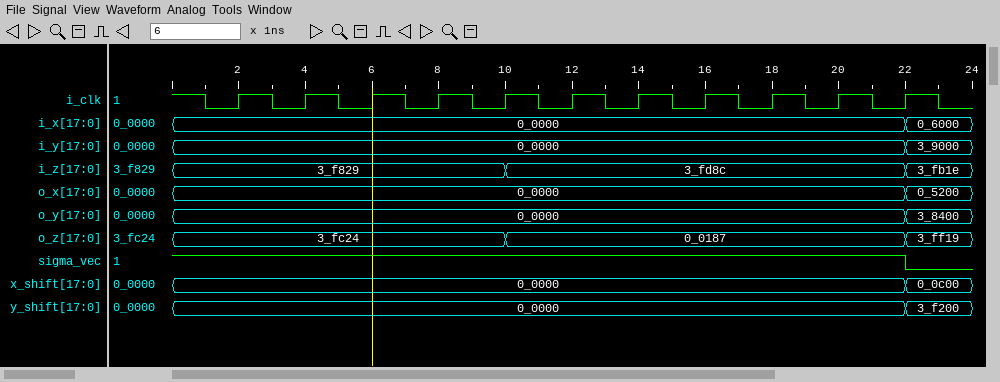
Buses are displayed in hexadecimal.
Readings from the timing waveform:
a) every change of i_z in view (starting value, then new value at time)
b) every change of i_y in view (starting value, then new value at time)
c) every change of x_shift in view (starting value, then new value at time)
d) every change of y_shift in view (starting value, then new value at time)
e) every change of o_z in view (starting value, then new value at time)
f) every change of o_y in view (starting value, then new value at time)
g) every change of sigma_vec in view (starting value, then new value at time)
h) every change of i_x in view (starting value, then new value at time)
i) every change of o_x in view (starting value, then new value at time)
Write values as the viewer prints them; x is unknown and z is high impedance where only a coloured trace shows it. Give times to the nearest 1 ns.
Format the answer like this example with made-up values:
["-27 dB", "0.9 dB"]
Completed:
["3_f829, 3_fd8c at 10 ns, 3_fb1e at 22 ns", "0_0000, 3_9000 at 22 ns", "0_0000, 0_0c00 at 22 ns", "0_0000, 3_f200 at 22 ns", "3_fc24, 0_0187 at 10 ns, 3_ff19 at 22 ns", "0_0000, 3_8400 at 22 ns", "1, 0 at 22 ns", "0_0000, 0_6000 at 22 ns", "0_0000, 0_5200 at 22 ns"]
